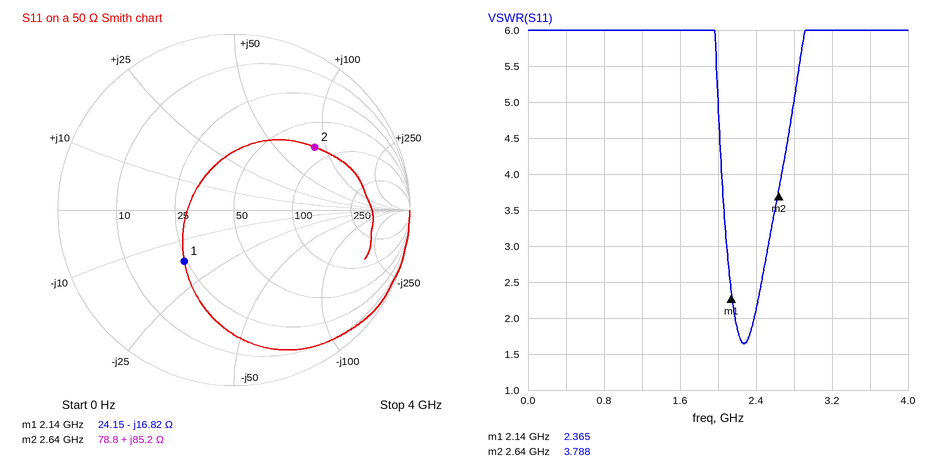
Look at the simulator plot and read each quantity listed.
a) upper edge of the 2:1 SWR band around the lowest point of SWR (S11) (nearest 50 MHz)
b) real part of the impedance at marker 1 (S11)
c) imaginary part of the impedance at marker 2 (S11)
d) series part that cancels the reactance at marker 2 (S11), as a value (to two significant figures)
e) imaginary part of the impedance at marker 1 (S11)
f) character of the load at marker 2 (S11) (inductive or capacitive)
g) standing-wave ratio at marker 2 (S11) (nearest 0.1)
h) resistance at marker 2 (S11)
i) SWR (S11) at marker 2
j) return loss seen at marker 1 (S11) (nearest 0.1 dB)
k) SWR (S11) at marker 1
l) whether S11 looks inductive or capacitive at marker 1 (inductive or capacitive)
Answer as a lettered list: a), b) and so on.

a) 2.40 GHz
b) 24.15 Ω
c) +85.2 Ω
d) 710 fF
e) -16.82 Ω
f) inductive
g) 3.8
h) 78.8 Ω
i) 3.788
j) 7.8 dB
k) 2.365
l) capacitive
